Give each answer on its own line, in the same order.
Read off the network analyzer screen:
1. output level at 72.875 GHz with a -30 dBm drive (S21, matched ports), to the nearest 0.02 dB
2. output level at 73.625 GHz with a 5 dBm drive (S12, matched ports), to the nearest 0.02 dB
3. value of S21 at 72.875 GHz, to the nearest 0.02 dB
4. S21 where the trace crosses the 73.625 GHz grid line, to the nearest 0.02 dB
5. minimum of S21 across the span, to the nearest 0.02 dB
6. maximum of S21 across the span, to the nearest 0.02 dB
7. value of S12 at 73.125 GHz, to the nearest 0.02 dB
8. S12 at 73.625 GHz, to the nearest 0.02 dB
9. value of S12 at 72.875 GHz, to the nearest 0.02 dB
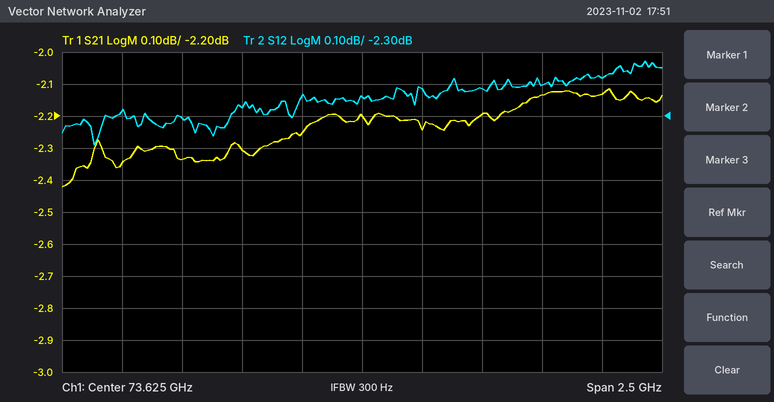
-32.34 dBm
2.76 dBm
-2.34 dB
-2.20 dB
-2.42 dB
-2.12 dB
-2.28 dB
-2.24 dB
-2.30 dB
